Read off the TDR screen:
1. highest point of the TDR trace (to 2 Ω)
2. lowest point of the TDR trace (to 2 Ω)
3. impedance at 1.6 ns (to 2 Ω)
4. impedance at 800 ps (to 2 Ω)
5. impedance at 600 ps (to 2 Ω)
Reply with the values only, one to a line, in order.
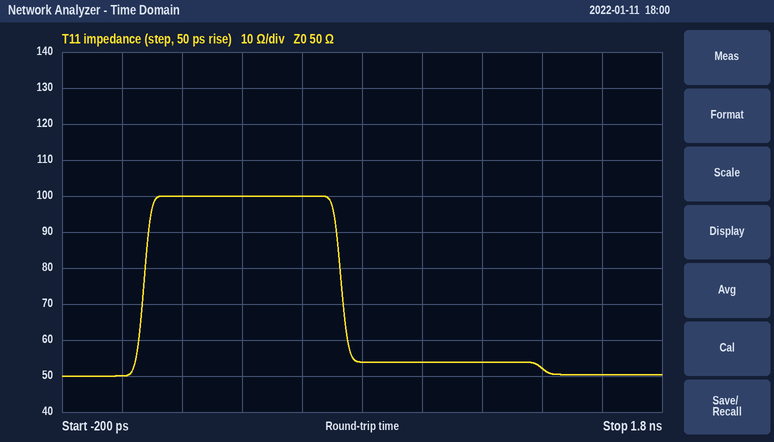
100 Ω
50 Ω
50 Ω
54 Ω
100 Ω
